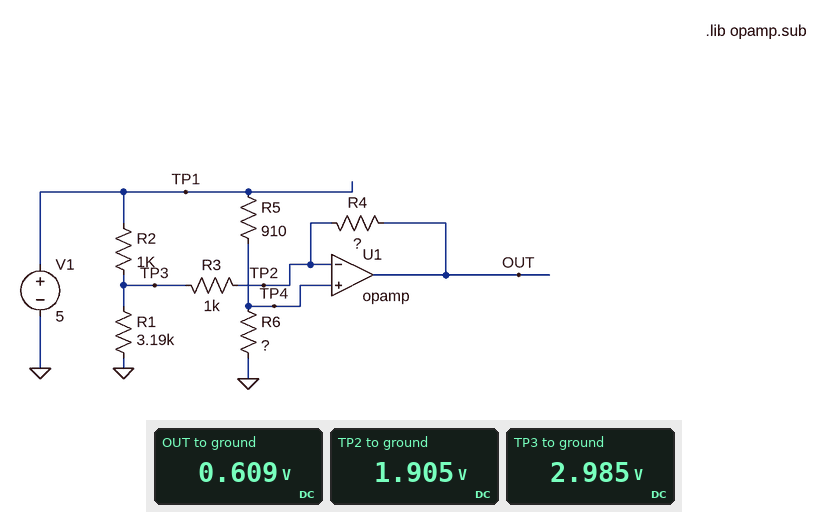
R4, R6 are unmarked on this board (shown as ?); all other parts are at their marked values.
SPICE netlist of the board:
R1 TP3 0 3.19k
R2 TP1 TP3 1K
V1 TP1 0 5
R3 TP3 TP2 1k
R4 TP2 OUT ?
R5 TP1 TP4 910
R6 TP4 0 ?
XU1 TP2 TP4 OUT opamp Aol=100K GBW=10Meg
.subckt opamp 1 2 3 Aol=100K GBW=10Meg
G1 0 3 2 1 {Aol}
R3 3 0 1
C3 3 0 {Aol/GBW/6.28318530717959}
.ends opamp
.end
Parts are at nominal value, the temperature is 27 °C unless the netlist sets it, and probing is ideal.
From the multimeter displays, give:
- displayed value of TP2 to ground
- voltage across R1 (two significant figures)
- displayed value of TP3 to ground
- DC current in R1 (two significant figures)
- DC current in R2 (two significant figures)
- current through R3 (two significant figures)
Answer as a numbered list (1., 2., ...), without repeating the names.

1. 1.905 V
2. 3.0 V
3. 2.985 V
4. 940 µA
5. 2.0 mA
6. 1.1 mA
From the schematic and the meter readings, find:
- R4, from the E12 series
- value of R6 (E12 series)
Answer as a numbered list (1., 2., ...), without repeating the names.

1. 1.2 kΩ
2. 560 Ω
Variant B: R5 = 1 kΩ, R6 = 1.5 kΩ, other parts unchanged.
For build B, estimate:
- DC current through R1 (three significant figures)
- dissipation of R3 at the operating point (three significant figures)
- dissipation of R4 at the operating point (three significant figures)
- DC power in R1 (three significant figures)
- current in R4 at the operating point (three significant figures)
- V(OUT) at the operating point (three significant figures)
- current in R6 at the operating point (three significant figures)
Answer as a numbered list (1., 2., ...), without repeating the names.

1. 1.08 mA
2. 210 µW
3. 252 µW
4. 3.75 mW
5. 458 µA
6. 2.45 V
7. 2.00 mA
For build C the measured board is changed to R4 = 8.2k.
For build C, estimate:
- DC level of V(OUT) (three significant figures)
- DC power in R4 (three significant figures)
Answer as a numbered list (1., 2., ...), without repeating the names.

1. -6.95 V
2. 9.56 mW
